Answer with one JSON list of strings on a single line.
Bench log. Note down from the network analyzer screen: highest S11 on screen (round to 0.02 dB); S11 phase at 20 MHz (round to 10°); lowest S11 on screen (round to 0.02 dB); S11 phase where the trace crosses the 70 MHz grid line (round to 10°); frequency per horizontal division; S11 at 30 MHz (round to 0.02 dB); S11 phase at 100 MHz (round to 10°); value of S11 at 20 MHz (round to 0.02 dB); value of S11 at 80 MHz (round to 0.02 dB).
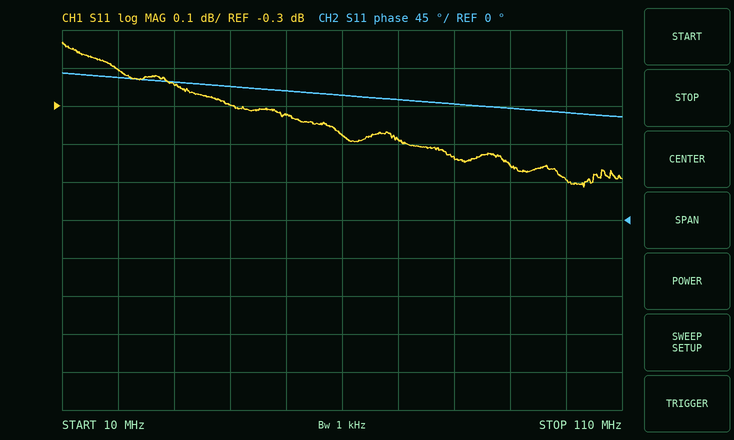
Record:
["-0.14 dB", "170°", "-0.52 dB", "140°", "10 MHz", "-0.24 dB", "130°", "-0.20 dB", "-0.44 dB"]
